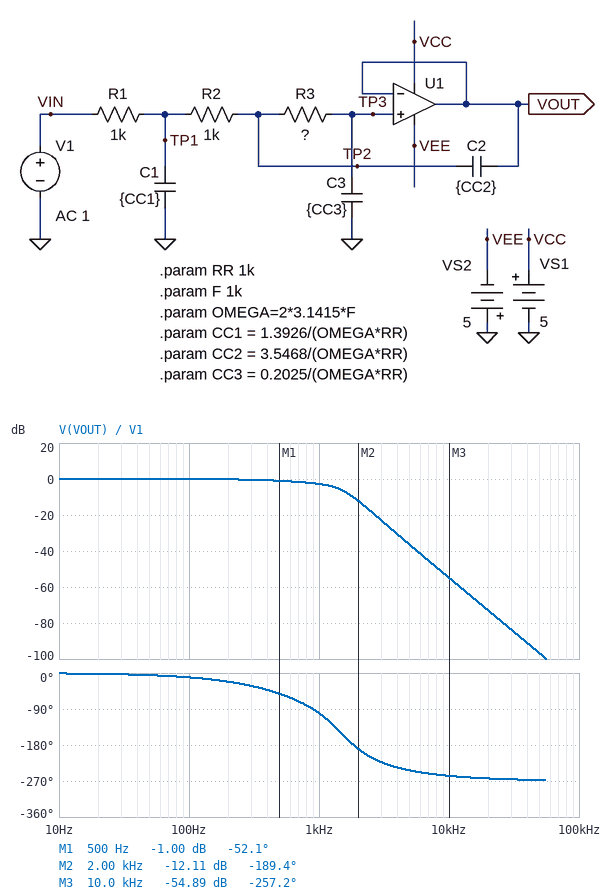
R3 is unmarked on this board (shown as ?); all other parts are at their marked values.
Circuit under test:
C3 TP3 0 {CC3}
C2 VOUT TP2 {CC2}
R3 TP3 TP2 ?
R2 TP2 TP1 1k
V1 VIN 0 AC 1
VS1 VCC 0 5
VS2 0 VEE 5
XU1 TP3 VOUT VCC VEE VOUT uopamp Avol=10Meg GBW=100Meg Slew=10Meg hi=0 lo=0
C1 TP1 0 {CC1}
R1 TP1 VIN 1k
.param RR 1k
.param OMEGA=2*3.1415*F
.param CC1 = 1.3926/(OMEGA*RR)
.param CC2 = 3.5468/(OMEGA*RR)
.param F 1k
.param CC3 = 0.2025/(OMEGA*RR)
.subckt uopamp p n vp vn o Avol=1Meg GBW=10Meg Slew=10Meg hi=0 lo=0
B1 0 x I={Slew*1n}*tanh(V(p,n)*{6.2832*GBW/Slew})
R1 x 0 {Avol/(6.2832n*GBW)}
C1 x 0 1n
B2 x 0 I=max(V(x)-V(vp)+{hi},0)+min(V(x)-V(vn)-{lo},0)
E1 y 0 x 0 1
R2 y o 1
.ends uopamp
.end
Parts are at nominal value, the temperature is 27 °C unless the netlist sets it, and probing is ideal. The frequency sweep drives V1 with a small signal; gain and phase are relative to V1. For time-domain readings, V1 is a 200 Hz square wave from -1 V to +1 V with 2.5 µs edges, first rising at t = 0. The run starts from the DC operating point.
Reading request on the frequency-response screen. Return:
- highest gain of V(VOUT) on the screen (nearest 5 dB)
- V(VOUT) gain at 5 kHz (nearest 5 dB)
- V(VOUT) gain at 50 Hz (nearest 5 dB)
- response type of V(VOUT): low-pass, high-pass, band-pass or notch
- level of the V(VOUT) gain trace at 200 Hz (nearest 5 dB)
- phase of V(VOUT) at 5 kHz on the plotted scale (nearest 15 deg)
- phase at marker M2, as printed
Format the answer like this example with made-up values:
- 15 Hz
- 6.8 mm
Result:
- 0 dB
- -35 dB
- 0 dB
- low-pass
- 0 dB
- -240 deg
- -189.4 deg
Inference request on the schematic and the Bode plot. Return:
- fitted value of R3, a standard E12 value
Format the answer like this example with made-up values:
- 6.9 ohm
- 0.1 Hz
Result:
- 560 Ω
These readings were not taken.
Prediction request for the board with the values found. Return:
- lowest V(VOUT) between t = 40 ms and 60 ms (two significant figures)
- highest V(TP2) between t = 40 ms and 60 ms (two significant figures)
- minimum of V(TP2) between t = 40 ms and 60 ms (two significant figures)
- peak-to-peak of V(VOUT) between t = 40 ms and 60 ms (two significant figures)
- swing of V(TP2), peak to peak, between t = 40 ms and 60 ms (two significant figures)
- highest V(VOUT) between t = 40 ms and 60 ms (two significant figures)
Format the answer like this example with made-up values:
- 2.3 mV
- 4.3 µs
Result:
- -1.0 V
- 1.0 V
- -1.0 V
- 2.0 V
- 2.0 V
- 1.0 V
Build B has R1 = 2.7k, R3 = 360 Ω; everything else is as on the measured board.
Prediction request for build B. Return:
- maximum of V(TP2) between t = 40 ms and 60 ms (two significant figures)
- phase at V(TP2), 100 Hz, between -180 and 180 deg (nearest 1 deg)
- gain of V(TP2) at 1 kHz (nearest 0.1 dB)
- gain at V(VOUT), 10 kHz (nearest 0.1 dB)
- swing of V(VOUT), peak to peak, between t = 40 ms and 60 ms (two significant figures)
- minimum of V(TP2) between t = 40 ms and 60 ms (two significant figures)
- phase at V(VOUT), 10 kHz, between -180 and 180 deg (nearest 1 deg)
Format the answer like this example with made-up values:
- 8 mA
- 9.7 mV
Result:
- 950 mV
- -25 deg
- -11.4 dB
- -59.5 dB
- 1.9 V
- -950 mV
- 102 deg
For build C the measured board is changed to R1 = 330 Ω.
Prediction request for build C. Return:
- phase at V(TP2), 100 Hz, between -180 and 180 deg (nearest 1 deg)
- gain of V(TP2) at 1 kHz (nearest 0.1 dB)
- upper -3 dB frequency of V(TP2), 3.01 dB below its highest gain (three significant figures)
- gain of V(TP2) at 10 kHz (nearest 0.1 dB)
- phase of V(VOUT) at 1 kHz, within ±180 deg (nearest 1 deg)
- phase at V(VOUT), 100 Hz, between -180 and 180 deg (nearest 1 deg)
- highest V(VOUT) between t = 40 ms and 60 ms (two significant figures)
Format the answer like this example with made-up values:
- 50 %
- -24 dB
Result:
- -4 deg
- 2.8 dB
- 1.63 kHz
- -41.9 dB
- -64 deg
- -5 deg
- 1.6 V
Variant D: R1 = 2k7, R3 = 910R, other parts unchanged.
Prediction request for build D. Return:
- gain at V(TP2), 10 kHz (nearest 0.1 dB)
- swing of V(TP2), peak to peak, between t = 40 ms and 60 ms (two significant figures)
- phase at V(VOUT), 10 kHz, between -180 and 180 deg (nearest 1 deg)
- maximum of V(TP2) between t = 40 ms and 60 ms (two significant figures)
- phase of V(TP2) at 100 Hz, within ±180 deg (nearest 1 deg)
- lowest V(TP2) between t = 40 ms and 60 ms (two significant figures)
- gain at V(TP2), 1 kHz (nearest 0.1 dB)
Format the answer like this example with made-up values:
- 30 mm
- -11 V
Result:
- -61.3 dB
- 1.9 V
- 99 deg
- 960 mV
- -25 deg
- -960 mV
- -11.1 dB
